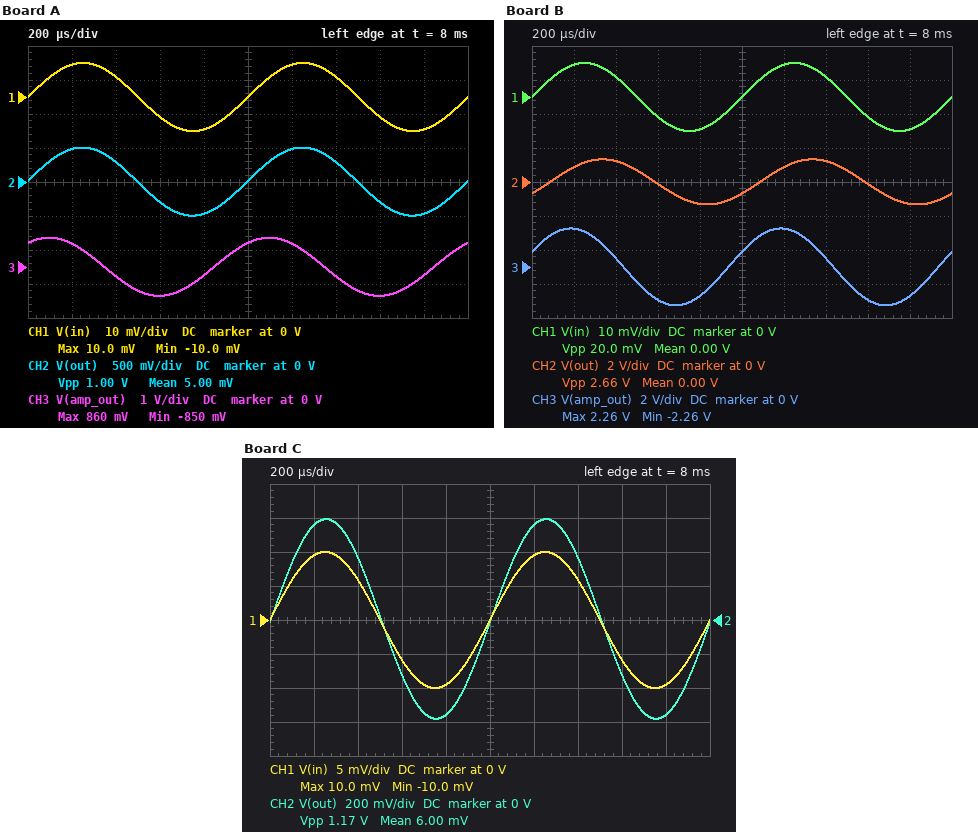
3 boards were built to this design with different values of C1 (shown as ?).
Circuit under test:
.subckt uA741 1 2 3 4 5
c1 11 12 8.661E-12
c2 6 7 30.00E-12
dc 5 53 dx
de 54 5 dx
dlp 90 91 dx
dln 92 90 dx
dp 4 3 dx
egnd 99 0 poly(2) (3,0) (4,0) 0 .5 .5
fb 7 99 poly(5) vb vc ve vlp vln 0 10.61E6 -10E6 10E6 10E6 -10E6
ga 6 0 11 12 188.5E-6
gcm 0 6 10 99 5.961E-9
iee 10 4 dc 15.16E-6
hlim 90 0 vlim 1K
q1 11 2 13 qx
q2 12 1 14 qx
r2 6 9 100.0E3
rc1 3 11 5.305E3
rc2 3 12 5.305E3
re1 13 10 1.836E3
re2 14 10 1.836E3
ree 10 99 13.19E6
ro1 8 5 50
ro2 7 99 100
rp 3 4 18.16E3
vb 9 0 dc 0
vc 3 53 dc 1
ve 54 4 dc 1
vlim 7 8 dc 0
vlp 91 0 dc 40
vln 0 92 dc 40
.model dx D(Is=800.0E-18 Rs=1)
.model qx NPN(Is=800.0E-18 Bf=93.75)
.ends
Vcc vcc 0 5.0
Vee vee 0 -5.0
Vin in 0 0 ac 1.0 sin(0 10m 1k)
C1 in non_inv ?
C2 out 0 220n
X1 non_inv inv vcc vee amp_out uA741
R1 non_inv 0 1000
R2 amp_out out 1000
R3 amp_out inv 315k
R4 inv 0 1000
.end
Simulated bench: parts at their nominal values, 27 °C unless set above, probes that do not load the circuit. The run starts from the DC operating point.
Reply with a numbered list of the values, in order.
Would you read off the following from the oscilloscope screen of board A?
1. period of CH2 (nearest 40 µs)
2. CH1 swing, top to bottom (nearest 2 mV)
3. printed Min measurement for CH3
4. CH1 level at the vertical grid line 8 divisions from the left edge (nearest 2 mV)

1. 1.00 ms
2. 20 mV
3. -850 mV
4. -6 mV
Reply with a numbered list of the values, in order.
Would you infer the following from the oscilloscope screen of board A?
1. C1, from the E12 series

1. 47 nF
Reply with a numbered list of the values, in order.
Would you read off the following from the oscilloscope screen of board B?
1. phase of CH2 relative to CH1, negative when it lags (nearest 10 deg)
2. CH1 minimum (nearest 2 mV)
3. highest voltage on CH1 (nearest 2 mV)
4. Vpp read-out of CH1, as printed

1. -30 deg
2. -10 mV
3. 10 mV
4. 20.0 mV
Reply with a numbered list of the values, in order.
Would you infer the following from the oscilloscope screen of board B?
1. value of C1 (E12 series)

1. 180 nF
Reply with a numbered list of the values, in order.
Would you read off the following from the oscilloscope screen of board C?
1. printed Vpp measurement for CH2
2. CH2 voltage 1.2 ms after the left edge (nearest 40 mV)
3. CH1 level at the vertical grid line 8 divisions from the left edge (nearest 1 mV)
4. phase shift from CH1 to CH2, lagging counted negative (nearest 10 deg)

1. 1.17 V
2. 560 mV
3. -6 mV
4. 0 deg
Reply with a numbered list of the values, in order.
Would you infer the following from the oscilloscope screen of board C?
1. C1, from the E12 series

1. 56 nF
